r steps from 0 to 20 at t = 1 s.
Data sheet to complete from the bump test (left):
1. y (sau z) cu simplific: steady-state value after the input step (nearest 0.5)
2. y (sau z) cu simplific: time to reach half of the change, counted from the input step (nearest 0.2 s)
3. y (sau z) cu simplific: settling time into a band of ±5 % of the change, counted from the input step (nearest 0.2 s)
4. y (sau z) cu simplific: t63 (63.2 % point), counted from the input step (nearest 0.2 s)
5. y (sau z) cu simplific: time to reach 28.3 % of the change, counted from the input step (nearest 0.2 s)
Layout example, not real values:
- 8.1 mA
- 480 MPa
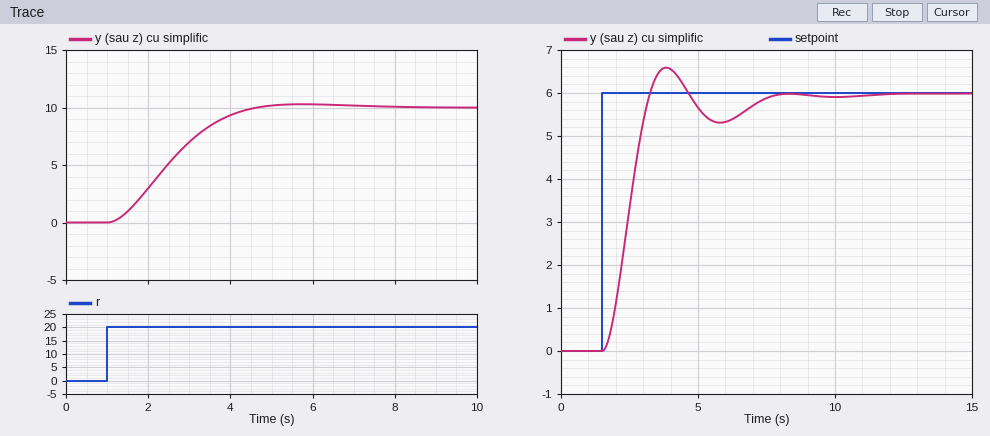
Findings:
- 10.0
- 1.4 s
- 3.2 s
- 1.8 s
- 1.0 s
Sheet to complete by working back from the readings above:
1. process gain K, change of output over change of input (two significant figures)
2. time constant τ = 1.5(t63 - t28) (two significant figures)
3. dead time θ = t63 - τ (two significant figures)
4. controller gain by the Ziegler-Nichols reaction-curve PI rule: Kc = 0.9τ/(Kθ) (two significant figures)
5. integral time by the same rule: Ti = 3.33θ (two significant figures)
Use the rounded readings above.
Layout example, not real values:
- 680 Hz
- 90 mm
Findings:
- 0.50
- 1.2 s
- 0.60 s
- 3.6
- 2.0 s
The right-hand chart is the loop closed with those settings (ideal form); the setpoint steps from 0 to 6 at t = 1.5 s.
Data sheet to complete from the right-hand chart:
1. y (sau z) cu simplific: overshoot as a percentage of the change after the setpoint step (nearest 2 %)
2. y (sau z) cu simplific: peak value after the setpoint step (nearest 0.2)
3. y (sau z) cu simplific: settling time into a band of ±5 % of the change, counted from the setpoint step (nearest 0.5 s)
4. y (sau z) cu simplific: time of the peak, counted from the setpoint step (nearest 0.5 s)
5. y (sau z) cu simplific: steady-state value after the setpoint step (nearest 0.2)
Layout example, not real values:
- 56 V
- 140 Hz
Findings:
- 10 %
- 6.6
- 5.5 s
- 2.5 s
- 6.0
